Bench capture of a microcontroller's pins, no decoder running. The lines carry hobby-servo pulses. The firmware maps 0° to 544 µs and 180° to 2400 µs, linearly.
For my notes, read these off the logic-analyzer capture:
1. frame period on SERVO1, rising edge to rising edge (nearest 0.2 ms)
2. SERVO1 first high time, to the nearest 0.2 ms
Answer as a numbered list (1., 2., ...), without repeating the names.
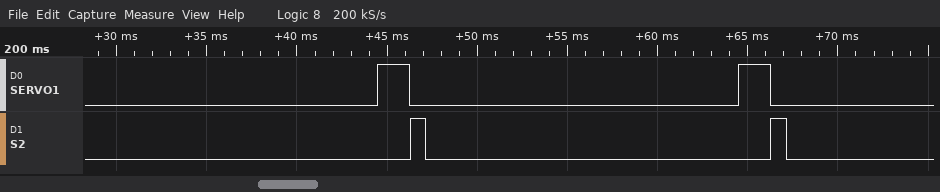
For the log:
1. 20.0 ms
2. 1.8 ms
